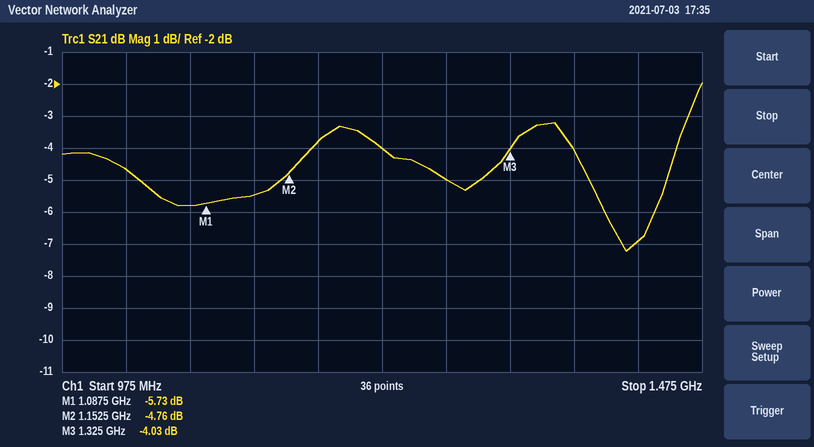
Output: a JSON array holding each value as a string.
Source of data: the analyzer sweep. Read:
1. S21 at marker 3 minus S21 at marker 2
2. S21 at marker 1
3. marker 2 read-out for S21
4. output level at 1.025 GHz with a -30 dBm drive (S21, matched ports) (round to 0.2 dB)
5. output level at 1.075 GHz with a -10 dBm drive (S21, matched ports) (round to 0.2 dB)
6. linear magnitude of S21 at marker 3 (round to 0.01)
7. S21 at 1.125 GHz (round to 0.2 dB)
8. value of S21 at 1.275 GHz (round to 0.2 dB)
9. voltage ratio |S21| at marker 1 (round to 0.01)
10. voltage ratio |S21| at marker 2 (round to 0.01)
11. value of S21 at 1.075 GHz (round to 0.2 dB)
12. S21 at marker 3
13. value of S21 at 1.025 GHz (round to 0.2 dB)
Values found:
["0.73 dB", "-5.73 dB", "-4.76 dB", "-34.6 dBm", "-15.8 dBm", "0.63", "-5.4 dB", "-5.0 dB", "0.52", "0.58", "-5.8 dB", "-4.03 dB", "-4.6 dB"]
